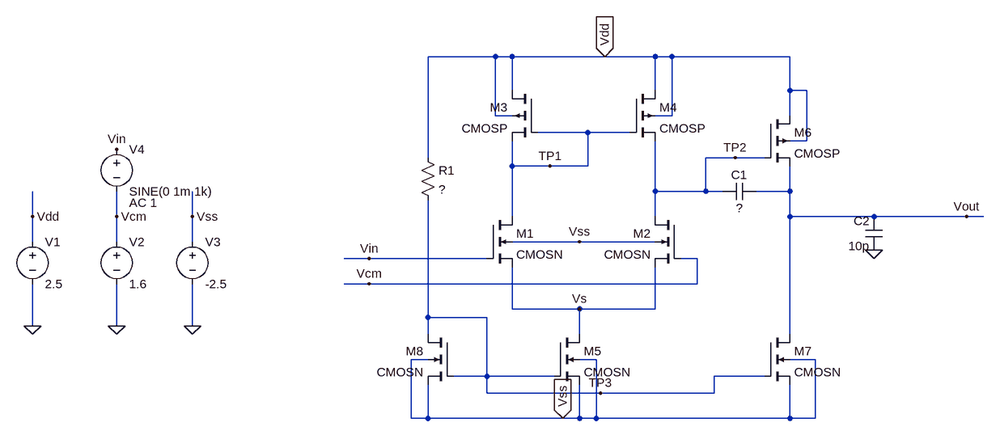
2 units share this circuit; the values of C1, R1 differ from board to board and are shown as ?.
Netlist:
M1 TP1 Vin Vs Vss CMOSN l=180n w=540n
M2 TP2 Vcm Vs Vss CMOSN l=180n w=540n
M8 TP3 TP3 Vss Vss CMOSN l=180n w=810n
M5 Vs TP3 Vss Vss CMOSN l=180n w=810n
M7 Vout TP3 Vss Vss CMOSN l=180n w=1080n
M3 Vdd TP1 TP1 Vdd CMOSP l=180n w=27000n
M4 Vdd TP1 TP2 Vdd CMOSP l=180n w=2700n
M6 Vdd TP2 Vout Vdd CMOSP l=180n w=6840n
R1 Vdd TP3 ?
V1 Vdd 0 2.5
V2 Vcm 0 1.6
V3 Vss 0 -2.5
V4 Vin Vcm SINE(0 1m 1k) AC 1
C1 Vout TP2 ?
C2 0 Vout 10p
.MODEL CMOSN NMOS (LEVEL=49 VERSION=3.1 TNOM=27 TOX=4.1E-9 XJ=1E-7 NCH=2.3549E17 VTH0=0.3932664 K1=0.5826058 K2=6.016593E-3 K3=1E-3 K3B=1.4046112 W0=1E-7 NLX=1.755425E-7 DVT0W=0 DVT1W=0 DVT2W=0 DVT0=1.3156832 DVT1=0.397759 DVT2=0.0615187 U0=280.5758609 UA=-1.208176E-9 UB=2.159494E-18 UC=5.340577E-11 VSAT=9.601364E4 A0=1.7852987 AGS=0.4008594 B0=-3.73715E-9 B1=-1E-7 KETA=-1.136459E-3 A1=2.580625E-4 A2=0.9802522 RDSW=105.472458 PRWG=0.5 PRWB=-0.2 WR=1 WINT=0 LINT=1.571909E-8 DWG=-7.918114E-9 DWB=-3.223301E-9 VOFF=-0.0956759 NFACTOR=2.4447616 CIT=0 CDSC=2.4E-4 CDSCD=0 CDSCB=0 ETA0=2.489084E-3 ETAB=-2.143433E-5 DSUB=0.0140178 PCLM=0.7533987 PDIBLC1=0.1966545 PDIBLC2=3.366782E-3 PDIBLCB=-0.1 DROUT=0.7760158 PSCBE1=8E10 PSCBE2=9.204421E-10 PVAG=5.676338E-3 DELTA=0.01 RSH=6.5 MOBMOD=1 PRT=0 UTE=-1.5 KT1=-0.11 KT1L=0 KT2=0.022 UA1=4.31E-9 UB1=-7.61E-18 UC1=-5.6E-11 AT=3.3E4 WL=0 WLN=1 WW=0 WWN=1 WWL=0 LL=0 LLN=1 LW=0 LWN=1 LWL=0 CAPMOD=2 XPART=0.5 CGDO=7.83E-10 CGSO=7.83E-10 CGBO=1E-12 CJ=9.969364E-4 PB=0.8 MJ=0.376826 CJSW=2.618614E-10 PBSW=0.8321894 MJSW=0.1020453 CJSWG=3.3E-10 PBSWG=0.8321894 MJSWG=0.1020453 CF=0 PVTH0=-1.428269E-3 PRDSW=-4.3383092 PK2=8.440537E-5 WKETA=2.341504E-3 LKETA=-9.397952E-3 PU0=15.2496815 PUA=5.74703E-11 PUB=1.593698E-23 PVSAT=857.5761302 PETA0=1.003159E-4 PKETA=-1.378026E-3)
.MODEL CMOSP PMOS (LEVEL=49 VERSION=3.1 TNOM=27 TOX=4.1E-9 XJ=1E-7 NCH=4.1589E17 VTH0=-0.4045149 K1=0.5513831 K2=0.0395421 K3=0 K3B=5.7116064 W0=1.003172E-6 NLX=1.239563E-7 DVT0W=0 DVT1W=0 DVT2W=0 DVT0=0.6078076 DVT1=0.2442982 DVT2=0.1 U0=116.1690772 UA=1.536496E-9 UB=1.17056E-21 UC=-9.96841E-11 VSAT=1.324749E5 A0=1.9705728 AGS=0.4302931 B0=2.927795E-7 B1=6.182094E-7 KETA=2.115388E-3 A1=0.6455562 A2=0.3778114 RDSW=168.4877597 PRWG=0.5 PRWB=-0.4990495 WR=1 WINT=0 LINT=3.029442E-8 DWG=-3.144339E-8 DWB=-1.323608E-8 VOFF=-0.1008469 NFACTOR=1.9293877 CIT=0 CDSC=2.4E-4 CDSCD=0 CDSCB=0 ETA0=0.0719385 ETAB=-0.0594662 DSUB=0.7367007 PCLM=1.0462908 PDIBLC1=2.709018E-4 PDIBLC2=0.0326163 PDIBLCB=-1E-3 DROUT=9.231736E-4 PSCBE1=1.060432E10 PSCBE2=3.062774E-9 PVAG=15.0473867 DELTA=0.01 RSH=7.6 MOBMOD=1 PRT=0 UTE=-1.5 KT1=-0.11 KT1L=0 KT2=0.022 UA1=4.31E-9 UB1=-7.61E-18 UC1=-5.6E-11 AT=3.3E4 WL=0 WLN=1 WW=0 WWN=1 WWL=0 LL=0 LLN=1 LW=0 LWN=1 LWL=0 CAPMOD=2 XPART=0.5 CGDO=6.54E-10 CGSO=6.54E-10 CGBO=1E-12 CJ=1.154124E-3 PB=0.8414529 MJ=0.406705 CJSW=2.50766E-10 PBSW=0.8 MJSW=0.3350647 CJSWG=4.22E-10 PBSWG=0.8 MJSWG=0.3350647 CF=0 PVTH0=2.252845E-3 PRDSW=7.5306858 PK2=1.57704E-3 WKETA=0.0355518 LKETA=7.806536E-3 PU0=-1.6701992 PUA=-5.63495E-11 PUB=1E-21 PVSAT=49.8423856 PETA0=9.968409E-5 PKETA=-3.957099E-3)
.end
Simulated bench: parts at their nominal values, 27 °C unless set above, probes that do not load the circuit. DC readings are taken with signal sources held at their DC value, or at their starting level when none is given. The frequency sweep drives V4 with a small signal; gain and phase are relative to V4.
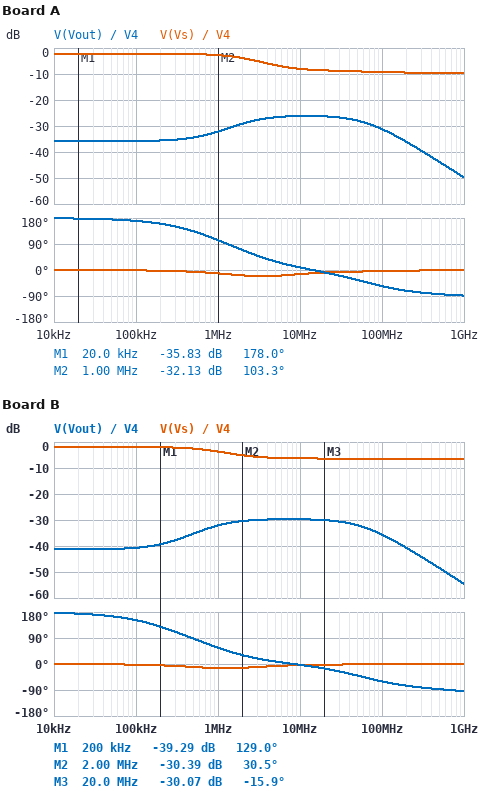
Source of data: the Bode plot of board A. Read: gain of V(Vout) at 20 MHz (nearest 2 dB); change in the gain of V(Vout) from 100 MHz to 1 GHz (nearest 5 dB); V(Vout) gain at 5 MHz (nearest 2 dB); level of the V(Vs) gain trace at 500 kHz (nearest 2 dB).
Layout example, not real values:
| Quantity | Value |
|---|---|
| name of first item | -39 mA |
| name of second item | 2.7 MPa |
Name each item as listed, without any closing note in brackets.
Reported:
| Quantity | Value |
|---|---|
| gain of V(Vout) at 20 MHz | -26 dB |
| change in the gain of V(Vout) from 100 MHz to 1 GHz | -20 dB |
| V(Vout) gain at 5 MHz | -26 dB |
| level of the V(Vs) gain trace at 500 kHz | -2 dB |
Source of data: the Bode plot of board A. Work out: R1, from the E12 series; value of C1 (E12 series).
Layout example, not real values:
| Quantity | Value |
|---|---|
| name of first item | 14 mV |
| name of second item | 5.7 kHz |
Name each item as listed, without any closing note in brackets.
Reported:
| Quantity | Value |
|---|---|
| R1, from the E12 series | 22 kΩ |
| value of C1 | 15 pF |
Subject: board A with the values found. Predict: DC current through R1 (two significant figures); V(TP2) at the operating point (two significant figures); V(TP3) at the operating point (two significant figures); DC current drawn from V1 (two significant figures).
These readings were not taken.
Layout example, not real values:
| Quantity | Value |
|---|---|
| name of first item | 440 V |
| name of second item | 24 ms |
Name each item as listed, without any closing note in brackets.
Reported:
| Quantity | Value |
|---|---|
| DC current through R1 | 180 µA |
| V(TP2) at the operating point | 14 mV |
| V(TP3) at the operating point | -1.4 V |
| DC current drawn from V1 | 700 µA |
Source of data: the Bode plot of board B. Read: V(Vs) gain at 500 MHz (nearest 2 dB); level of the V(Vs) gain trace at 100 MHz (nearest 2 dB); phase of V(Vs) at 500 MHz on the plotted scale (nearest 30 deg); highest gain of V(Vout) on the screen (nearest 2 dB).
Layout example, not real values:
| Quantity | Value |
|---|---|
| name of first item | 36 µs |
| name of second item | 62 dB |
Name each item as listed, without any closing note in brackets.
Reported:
| Quantity | Value |
|---|---|
| V(Vs) gain at 500 MHz | -6 dB |
| level of the V(Vs) gain trace at 100 MHz | -6 dB |
| phase of V(Vs) at 500 MHz on the plotted scale | 0 deg |
| highest gain of V(Vout) on the screen | -30 dB |
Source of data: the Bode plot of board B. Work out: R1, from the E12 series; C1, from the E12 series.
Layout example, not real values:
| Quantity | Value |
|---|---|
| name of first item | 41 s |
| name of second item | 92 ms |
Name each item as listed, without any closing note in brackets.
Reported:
| Quantity | Value |
|---|---|
| R1, from the E12 series | 150 kΩ |
| C1, from the E12 series | 18 pF |
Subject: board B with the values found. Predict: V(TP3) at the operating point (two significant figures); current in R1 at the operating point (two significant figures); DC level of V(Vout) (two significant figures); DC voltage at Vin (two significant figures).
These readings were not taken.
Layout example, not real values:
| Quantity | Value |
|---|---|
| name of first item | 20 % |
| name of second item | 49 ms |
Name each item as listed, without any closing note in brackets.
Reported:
| Quantity | Value |
|---|---|
| V(TP3) at the operating point | -1.8 V |
| current in R1 at the operating point | 29 µA |
| DC level of V(Vout) | 2.5 V |
| DC voltage at Vin | 1.6 V |
